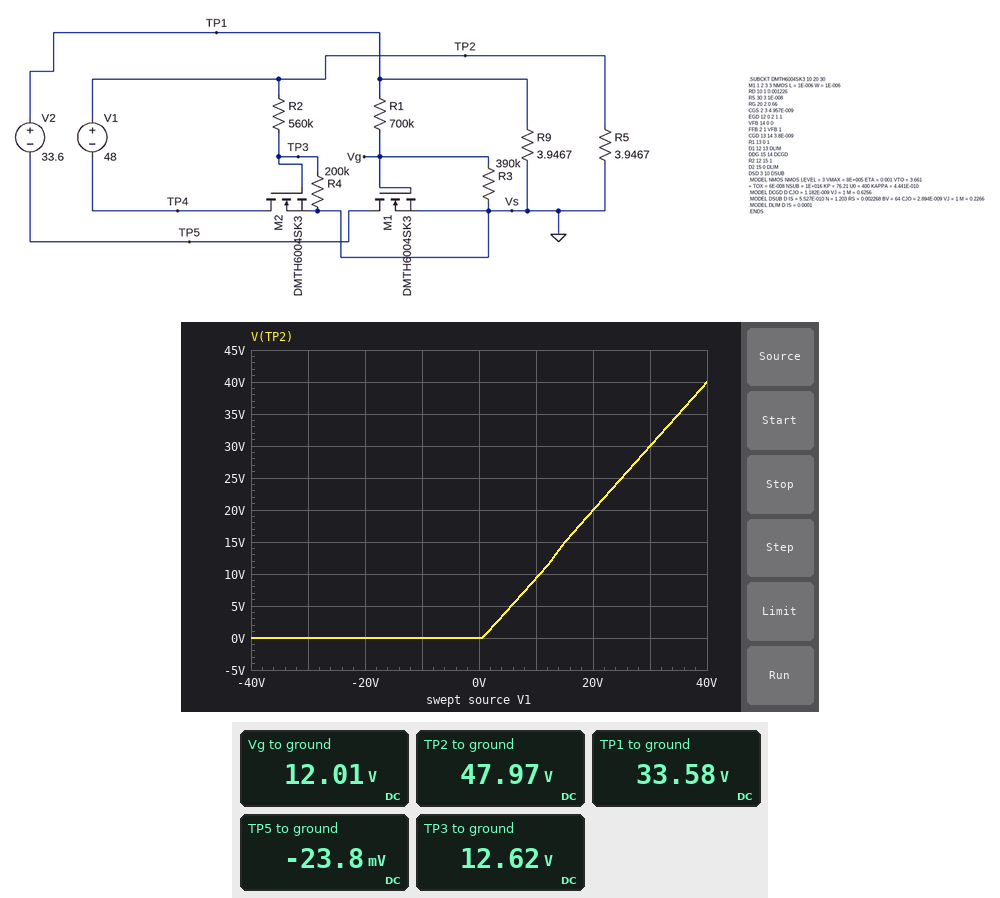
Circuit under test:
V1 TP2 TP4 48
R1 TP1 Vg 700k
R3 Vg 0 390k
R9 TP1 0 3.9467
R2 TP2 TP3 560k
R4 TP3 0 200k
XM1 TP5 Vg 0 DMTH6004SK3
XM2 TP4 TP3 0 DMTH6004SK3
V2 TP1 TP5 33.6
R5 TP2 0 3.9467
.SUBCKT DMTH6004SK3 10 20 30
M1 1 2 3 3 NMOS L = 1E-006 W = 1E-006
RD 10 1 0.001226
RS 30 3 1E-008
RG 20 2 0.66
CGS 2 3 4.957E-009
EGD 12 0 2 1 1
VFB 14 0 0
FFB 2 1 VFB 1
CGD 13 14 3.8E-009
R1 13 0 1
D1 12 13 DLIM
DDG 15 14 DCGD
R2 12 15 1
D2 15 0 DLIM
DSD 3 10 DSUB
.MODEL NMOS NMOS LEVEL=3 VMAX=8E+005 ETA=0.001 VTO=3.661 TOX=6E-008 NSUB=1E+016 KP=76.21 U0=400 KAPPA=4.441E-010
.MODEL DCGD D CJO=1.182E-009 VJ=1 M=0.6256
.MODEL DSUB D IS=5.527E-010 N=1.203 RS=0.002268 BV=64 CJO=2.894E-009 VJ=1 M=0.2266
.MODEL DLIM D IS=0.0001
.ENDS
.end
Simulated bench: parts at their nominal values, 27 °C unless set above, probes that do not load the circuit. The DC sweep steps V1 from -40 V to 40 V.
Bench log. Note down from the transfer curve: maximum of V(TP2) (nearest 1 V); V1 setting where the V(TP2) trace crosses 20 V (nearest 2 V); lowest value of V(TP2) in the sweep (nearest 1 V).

40 V
20 V
0 V
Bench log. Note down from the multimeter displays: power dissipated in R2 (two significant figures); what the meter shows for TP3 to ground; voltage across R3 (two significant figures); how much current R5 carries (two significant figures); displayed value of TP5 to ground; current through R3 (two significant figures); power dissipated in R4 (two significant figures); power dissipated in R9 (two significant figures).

2.2 mW
12.62 V
12 V
12 A
-23.8 mV
31 µA
800 µW
290 W
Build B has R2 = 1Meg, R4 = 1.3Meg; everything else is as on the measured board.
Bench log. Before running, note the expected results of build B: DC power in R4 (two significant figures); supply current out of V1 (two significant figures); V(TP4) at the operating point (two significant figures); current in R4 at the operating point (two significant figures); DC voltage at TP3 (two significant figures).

570 µW
12 A
-22 mV
21 µA
27 V
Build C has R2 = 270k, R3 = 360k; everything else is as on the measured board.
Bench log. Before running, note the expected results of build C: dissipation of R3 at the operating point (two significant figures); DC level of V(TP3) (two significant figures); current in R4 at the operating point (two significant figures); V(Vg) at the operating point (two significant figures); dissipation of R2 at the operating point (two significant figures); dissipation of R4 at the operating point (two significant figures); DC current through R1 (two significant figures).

360 µW
20 V
100 µA
11 V
2.8 mW
2.1 mW
32 µA
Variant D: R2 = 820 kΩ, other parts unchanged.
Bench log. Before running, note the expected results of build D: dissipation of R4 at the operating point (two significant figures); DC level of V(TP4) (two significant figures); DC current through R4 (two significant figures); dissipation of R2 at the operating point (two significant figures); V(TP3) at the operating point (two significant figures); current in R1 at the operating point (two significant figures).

440 µW
-43 mV
47 µA
1.8 mW
9.4 V
31 µA
